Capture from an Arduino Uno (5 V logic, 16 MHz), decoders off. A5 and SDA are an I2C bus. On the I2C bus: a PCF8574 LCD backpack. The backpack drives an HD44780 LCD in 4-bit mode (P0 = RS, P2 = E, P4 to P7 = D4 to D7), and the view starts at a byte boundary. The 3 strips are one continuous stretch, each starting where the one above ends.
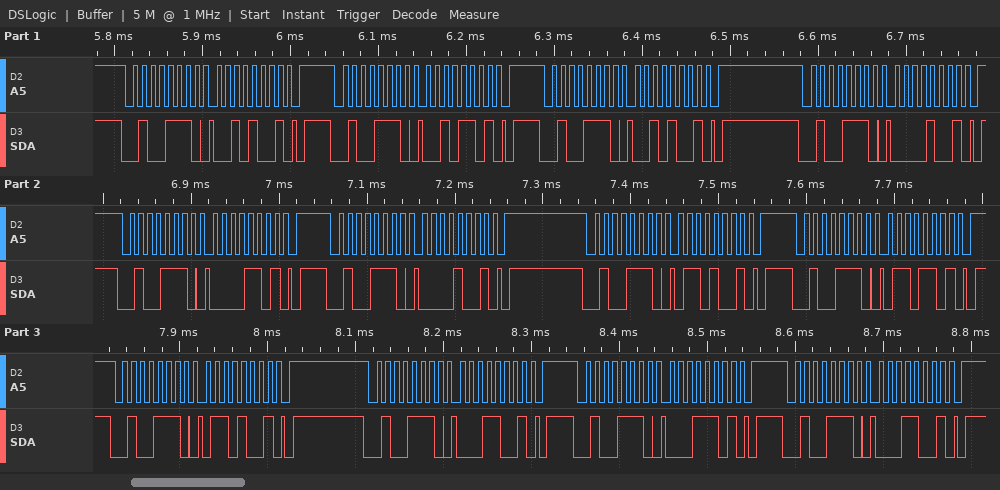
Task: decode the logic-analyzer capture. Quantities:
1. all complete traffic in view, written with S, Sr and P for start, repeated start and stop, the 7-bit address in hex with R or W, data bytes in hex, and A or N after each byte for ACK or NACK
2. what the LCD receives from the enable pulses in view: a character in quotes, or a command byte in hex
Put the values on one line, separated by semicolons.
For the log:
S 27W A 29 A P S 27W A 2D A P S 27W A 29 A P S 27W A 09 A P S 27W A 0D A P S 27W A 09 A P S 27W A 69 A P S 27W A 6D A P S 27W A 69 A P S 27W A 19 A P S 27W A 1D A P S 27W A 19 A P; ' ' 'a'
